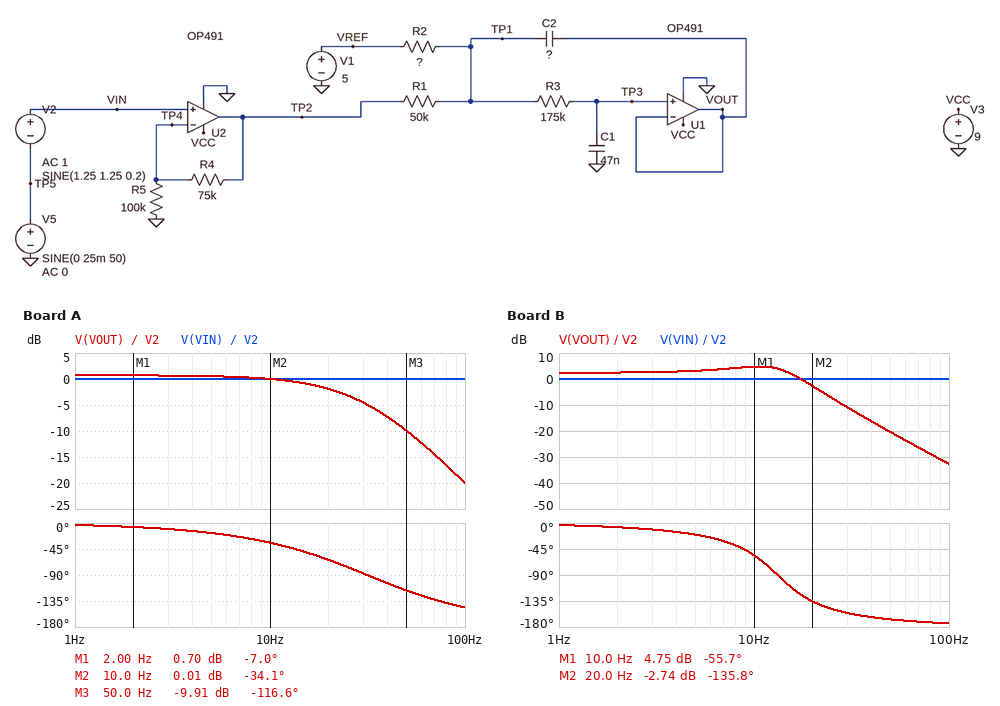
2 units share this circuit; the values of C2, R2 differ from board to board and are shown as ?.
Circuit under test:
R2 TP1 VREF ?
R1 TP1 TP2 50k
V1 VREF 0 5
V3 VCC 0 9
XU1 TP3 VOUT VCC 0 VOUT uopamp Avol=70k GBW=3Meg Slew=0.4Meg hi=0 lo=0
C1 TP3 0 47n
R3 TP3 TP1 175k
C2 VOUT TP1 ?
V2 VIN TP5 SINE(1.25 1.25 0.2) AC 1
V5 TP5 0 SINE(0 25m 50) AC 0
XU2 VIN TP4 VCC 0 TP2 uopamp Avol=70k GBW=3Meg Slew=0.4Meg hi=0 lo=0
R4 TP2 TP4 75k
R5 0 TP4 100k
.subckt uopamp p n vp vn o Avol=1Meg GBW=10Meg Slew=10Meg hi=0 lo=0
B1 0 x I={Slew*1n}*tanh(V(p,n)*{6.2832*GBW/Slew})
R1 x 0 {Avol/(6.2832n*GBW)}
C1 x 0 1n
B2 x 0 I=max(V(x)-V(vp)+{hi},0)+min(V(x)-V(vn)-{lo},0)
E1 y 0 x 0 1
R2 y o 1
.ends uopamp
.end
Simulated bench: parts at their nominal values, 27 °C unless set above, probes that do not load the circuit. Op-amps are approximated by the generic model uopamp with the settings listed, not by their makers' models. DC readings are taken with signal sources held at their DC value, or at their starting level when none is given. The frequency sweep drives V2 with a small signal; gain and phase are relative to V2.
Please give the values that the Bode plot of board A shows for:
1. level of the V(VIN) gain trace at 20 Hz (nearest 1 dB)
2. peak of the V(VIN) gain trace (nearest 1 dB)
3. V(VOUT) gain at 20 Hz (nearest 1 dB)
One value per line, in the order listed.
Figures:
0 dB
0 dB
-2 dB
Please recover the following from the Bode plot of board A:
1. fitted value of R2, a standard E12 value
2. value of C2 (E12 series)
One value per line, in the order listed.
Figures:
82 kΩ
100 nF
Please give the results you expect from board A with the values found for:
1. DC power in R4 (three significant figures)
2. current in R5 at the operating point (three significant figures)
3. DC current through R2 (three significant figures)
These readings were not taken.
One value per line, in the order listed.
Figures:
11.7 µW
12.5 µA
21.3 µA
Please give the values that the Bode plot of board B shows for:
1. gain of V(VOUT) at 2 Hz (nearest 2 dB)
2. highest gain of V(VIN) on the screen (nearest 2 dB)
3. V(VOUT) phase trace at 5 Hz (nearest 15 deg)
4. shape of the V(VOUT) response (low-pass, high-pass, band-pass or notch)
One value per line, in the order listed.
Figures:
2 dB
0 dB
-15 deg
low-pass
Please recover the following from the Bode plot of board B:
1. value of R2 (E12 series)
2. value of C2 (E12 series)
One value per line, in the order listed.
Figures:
150 kΩ
470 nF
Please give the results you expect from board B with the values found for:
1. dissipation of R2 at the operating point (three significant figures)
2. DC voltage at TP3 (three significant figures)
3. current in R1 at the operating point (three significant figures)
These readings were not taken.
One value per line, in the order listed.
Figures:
29.7 µW
2.89 V
14.1 µA
